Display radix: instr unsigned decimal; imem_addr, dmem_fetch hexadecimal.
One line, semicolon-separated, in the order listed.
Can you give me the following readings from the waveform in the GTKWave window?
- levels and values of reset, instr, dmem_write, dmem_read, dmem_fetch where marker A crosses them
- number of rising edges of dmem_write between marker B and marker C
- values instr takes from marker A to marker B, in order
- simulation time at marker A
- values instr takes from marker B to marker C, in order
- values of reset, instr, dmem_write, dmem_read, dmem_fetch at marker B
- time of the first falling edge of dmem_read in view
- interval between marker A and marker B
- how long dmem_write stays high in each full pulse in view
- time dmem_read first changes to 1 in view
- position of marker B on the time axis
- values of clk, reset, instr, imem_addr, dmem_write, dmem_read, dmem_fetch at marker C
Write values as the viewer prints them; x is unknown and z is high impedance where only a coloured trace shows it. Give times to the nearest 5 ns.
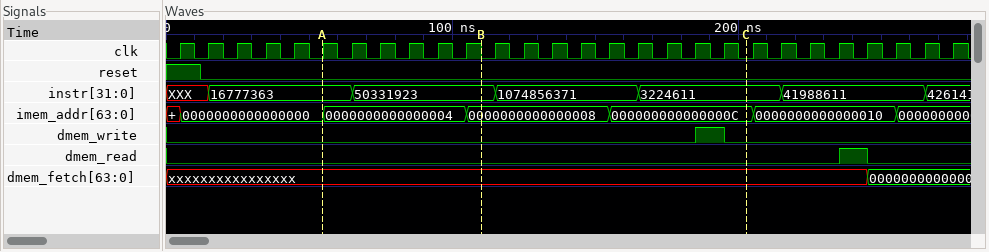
reset=0, instr=16777363, dmem_write=0, dmem_read=0, dmem_fetch=xxxxxxxxxxxxxxxx; 1; 16777363, 50331923; 55 ns; 50331923, 1074856371, 3224611; reset=0, instr=50331923, dmem_write=0, dmem_read=0, dmem_fetch=xxxxxxxxxxxxxxxx; 245 ns; 55 ns; 10 ns; 235 ns; 110 ns; clk=0, reset=0, instr=3224611, imem_addr=000000000000000C, dmem_write=0, dmem_read=0, dmem_fetch=xxxxxxxxxxxxxxxx
